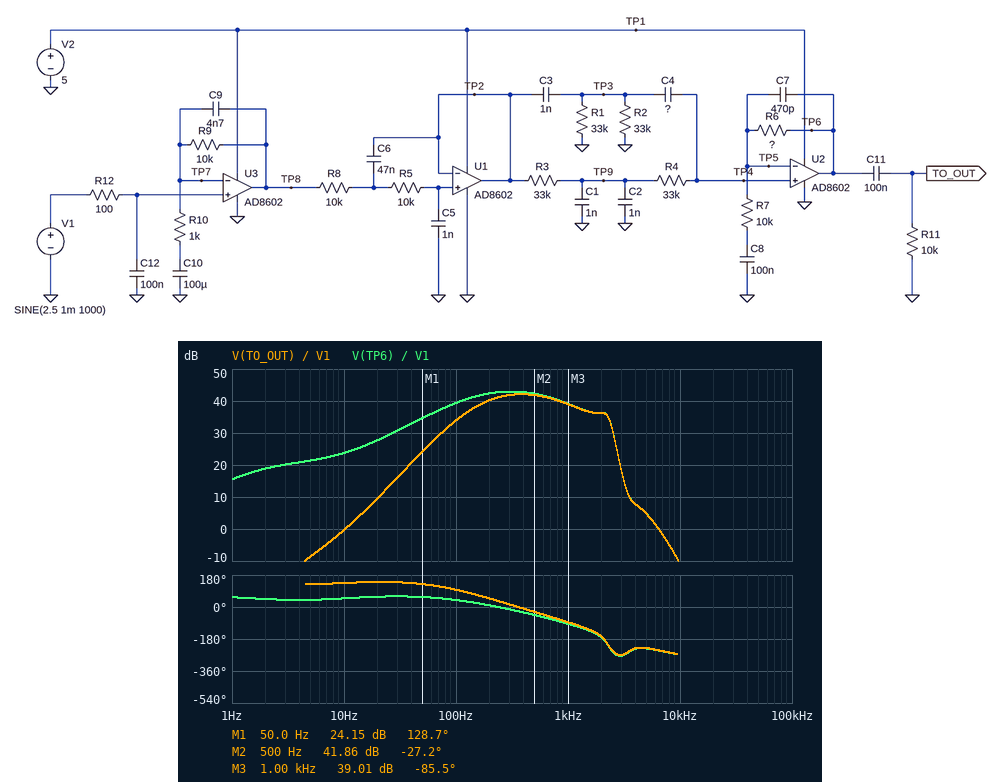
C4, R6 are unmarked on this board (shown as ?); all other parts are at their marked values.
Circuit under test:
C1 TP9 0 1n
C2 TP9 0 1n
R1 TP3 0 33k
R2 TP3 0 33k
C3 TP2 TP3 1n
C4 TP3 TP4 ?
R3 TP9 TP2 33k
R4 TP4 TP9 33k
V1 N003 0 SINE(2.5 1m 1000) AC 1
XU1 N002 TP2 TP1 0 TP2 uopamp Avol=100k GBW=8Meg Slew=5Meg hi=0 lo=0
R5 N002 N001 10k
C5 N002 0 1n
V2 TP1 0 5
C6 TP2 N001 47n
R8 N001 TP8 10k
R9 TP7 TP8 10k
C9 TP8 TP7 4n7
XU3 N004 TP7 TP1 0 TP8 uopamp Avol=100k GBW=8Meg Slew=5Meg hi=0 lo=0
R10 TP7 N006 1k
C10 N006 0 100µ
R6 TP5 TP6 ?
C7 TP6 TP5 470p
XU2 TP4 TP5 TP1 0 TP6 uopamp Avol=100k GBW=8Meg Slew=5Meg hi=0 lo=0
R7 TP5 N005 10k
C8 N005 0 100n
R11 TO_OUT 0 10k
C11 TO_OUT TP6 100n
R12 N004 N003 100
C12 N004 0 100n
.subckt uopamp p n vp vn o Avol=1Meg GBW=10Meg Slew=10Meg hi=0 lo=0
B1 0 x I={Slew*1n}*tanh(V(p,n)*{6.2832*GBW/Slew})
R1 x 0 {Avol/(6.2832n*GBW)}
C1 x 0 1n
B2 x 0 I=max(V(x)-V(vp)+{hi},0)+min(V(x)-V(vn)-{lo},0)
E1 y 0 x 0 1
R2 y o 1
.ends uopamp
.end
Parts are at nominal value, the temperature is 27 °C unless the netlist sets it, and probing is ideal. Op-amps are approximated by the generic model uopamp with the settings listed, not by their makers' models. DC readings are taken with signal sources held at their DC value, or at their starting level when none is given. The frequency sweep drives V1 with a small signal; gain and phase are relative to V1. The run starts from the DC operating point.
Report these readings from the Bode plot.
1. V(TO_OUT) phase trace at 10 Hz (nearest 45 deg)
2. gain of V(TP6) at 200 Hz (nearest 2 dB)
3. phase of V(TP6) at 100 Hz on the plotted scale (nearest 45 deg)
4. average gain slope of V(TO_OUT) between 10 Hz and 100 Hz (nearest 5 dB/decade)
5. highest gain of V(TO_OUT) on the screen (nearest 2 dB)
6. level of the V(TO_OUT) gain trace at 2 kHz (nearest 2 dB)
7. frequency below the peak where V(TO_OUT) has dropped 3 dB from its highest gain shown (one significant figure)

135 deg
42 dB
45 deg
35 dB/decade
42 dB
36 dB
200 Hz
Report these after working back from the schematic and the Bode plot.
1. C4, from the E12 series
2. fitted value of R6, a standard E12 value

2.7 nF
150 kΩ
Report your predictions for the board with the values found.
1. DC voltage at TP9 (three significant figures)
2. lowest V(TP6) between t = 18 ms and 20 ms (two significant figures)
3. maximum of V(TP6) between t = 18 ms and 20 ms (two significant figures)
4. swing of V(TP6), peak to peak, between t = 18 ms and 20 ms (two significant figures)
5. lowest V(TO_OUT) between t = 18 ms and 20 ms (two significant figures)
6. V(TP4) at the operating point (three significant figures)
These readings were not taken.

2.50 V
2.4 V
2.6 V
180 mV
-89 mV
2.50 V
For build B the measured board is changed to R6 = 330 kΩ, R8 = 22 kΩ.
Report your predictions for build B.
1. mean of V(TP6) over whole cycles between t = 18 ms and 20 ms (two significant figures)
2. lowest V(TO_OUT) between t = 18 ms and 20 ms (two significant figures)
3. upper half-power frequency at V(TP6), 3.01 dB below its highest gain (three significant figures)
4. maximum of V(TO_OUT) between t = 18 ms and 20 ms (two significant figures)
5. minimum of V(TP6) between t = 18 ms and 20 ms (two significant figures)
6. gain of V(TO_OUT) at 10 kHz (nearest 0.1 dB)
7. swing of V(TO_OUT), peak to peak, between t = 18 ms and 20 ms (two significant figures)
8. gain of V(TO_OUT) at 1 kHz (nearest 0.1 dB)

2.5 V
-200 mV
884 Hz
200 mV
2.3 V
-17.9 dB
390 mV
45.8 dB
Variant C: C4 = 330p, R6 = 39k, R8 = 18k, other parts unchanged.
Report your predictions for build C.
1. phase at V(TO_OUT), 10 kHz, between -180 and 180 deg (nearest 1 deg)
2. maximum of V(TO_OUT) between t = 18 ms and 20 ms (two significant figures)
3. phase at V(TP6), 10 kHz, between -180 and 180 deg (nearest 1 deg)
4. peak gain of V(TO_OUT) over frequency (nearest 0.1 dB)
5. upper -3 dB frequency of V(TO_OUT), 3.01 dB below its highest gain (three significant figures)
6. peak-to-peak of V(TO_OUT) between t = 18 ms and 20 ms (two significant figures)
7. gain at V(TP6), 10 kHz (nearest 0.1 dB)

159 deg
64 mV
158 deg
41.1 dB
1.89 kHz
130 mV
-25.7 dB
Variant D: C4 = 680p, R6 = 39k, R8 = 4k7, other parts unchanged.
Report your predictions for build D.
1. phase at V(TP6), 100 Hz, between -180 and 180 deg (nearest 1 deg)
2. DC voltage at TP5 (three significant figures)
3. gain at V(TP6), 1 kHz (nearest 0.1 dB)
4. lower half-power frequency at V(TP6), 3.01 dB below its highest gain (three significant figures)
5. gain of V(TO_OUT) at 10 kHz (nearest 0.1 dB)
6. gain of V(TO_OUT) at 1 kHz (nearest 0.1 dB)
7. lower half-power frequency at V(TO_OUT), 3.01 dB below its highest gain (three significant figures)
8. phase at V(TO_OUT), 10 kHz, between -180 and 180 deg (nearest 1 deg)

34 deg
2.50 V
33.1 dB
128 Hz
-7.8 dB
33.0 dB
201 Hz
140 deg
